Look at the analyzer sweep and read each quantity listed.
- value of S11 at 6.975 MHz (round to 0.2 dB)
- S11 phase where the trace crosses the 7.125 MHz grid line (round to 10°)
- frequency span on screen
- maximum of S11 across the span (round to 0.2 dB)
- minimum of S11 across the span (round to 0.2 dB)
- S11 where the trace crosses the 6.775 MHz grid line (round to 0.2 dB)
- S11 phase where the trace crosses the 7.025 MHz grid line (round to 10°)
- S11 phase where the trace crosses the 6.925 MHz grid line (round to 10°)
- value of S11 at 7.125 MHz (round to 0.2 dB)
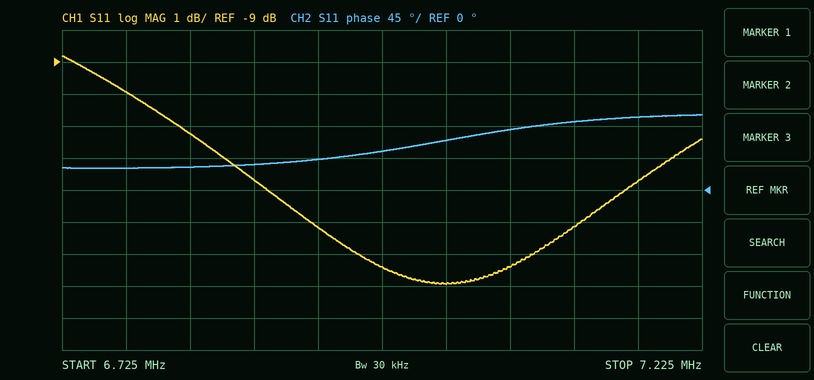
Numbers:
-15.4 dB
100°
500 kHz
-8.8 dB
-16.0 dB
-10.0 dB
70°
40°
-14.2 dB
